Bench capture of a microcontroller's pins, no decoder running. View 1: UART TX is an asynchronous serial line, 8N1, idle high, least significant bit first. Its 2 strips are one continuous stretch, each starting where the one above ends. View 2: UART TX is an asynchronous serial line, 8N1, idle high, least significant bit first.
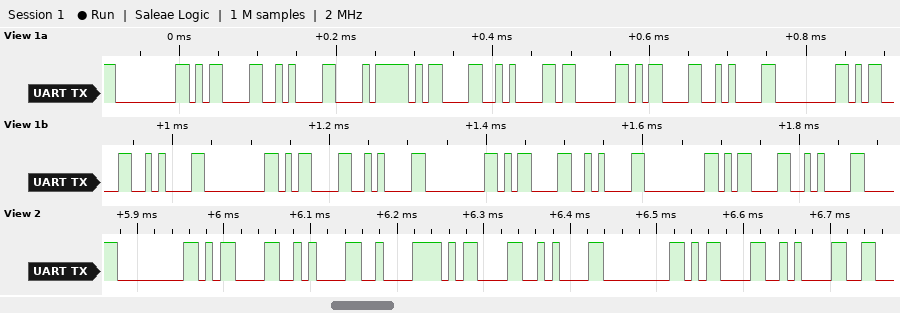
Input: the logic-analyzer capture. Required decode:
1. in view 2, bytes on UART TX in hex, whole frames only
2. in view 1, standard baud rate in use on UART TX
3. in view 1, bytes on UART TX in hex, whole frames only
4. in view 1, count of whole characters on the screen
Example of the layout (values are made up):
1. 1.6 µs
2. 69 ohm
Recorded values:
1. 00 0D 0A C2 0D 0A 00 0D 0A
2. 115200 baud
3. 00 0D 0A E8 0D 0A 03 0D 0A 00 0D 0A 00 0D 0A 00 0D 0A 00 0D 0A
4. 21
